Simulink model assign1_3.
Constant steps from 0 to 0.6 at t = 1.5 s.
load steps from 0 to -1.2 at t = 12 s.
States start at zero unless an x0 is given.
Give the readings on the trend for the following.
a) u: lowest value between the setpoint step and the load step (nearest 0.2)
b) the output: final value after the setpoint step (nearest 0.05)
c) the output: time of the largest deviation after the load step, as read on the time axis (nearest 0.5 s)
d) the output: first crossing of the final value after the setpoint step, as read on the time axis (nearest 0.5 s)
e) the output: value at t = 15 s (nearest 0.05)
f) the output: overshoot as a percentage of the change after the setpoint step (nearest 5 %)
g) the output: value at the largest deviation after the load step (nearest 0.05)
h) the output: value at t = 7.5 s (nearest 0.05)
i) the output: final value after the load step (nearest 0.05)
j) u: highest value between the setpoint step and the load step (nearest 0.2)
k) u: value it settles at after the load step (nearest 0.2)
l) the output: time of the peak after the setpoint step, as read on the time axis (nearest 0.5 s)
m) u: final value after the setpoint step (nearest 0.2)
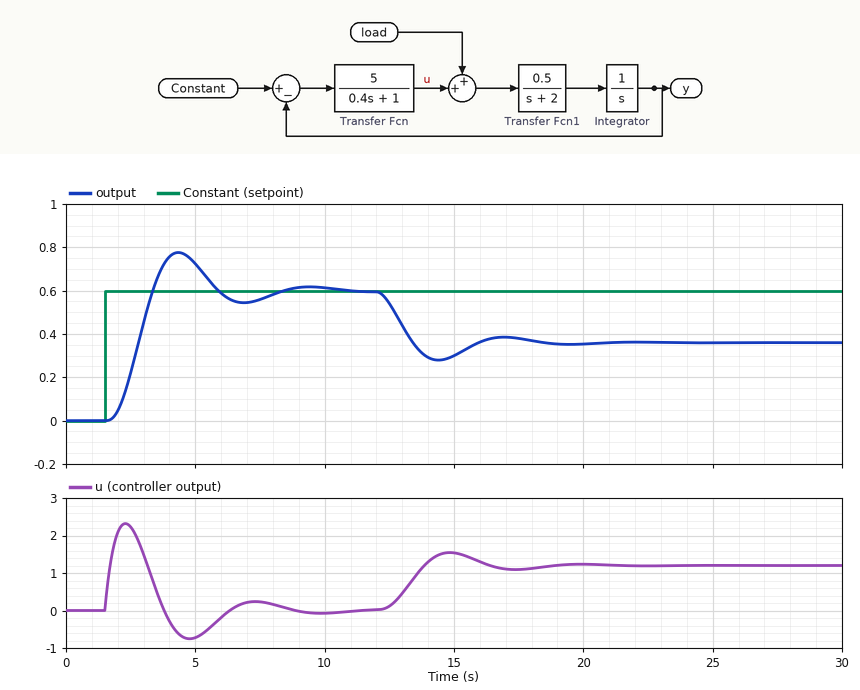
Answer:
-0.8
0.60
14.5 s
3.5 s
0.30
30 %
0.30
0.55
0.35
2.4
1.2
4.5 s
0.0
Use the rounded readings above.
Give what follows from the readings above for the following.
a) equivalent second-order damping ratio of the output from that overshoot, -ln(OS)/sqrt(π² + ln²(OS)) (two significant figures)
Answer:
0.36
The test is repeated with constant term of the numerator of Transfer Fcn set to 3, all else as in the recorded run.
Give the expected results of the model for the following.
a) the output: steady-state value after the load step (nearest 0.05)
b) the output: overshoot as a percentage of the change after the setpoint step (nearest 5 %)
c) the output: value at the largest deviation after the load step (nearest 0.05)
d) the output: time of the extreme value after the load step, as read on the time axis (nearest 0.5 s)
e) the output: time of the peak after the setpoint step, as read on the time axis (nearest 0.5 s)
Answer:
0.20
10 %
0.15
15.5 s
5.5 s
